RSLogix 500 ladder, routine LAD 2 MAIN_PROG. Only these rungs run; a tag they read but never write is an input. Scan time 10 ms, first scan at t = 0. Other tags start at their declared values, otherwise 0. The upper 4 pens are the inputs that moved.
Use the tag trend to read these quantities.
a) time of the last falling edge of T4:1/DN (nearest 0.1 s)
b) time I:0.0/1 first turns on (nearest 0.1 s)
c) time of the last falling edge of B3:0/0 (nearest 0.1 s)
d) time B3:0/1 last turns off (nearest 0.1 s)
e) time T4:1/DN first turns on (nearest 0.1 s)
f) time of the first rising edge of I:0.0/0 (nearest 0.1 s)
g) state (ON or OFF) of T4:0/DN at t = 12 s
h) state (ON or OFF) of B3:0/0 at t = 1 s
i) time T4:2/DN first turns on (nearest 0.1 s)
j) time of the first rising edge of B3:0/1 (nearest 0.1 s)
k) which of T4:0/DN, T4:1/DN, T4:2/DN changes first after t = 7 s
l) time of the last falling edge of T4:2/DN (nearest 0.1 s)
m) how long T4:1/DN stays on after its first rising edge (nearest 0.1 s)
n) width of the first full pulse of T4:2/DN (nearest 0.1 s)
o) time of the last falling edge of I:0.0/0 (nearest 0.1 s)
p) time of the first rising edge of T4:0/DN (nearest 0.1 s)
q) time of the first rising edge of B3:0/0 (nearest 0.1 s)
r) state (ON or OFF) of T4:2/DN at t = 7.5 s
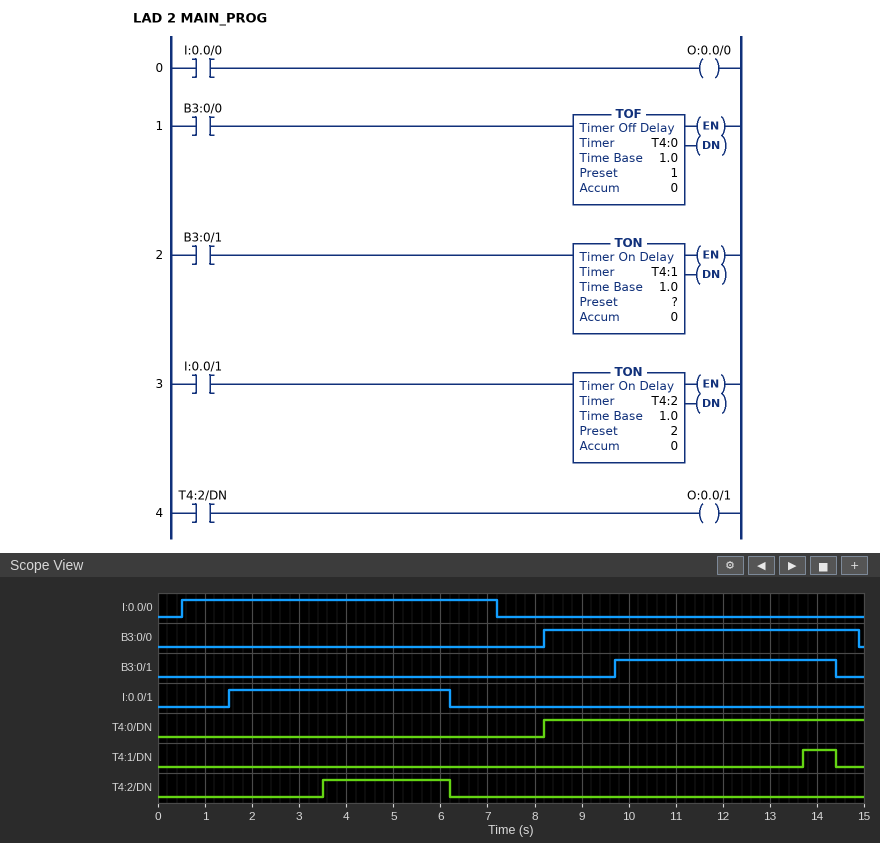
14.4 s
1.5 s
14.9 s
14.4 s
13.7 s
0.5 s
ON
OFF
3.5 s
9.7 s
T4:0/DN
6.2 s
0.7 s
2.7 s
7.2 s
8.2 s
8.2 s
OFF
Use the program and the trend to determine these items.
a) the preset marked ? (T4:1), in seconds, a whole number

4 s
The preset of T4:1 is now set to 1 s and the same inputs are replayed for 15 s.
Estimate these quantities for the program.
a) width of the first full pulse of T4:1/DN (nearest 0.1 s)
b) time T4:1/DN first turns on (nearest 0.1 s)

3.7 s
10.7 s
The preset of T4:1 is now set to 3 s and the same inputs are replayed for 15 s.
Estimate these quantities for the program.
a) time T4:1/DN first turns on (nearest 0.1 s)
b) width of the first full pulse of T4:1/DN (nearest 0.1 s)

12.7 s
1.7 s
